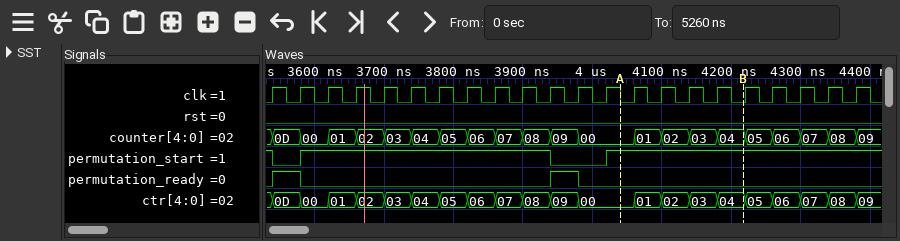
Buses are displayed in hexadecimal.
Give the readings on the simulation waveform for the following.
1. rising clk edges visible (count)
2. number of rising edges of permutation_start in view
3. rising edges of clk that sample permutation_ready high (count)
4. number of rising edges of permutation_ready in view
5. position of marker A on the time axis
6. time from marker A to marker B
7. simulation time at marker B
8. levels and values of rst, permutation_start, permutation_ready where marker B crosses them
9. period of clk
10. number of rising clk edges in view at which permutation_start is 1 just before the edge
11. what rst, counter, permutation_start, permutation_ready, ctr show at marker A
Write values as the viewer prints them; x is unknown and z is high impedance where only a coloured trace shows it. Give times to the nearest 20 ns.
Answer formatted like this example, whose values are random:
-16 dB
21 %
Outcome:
22
2
2
2
4040 ns
180 ns
4220 ns
rst=0, permutation_start=1, permutation_ready=0
40 ns
19
rst=0, counter=00, permutation_start=1, permutation_ready=0, ctr=00
